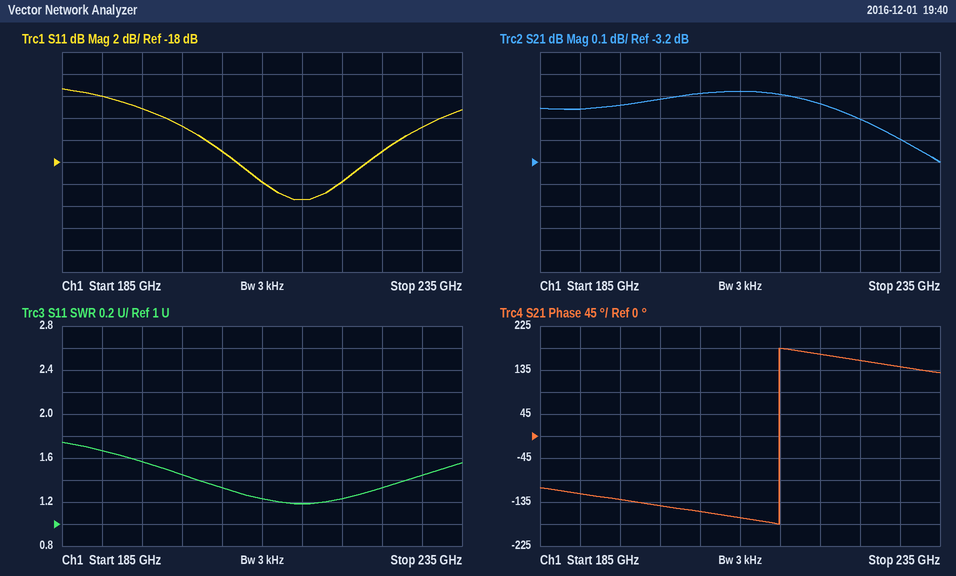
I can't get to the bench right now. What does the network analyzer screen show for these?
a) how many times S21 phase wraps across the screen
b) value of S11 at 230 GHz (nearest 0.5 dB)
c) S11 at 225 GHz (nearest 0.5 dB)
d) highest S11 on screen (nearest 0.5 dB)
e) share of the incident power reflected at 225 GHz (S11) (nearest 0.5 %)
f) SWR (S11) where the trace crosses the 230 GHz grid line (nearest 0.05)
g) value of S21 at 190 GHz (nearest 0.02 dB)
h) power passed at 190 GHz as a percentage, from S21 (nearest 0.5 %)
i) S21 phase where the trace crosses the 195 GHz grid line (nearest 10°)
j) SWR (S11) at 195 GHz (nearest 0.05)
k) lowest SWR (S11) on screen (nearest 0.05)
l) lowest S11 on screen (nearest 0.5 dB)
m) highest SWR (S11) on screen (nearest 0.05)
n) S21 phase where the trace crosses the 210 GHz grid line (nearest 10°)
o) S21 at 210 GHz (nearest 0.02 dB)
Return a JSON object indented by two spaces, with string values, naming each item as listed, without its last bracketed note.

{
  "how many times S21 phase wraps across the screen": "1",
  "value of S11 at 230 GHz": "-15.0 dB",
  "S11 at 225 GHz": "-17.0 dB",
  "highest S11 on screen": "-11.5 dB",
  "share of the incident power reflected at 225 GHz (S11)": "2.0 %",
  "SWR (S11) where the trace crosses the 230 GHz grid line": "1.45",
  "value of S21 at 190 GHz": "-2.96 dB",
  "power passed at 190 GHz as a percentage, from S21": "50.5 %",
  "S21 phase where the trace crosses the 195 GHz grid line": "-130°",
  "SWR (S11) at 195 GHz": "1.55",
  "lowest SWR (S11) on screen": "1.20",
  "lowest S11 on screen": "-21.5 dB",
  "highest SWR (S11) on screen": "1.75",
  "S21 phase where the trace crosses the 210 GHz grid line": "-170°",
  "S21 at 210 GHz": "-2.88 dB"
}
